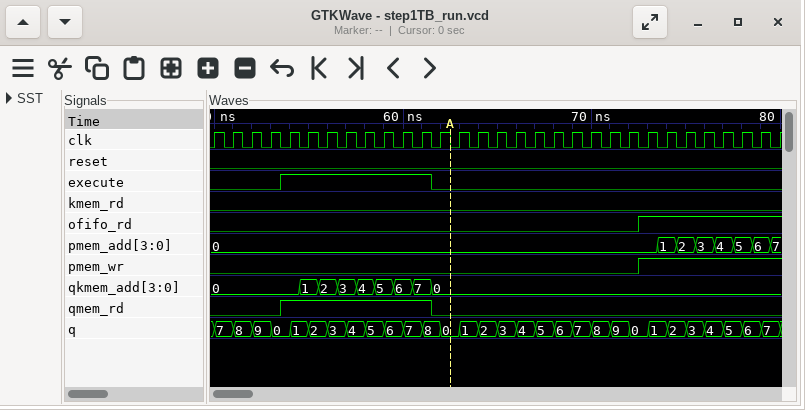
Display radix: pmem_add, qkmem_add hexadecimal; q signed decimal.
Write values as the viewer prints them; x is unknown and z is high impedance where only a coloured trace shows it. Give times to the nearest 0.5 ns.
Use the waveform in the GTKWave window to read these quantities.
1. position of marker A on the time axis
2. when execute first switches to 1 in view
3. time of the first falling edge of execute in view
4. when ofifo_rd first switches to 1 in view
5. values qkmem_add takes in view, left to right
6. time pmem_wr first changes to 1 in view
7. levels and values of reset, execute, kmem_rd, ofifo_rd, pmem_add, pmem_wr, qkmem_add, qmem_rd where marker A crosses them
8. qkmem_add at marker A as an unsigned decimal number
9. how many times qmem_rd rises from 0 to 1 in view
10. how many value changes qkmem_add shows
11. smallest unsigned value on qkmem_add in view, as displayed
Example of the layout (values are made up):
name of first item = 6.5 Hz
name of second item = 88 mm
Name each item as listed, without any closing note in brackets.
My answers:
position of marker A on the time axis = 62.5 ns
when execute first switches to 1 in view = 53.5 ns
time of the first falling edge of execute in view = 61.5 ns
when ofifo_rd first switches to 1 in view = 72.5 ns
values qkmem_add takes in view, left to right = 0, 1, 2, 3, 4, 5, 6, 7, 0
time pmem_wr first changes to 1 in view = 72.5 ns
levels and values of reset, execute, kmem_rd, ofifo_rd, pmem_add, pmem_wr, qkmem_add, qmem_rd where marker A crosses them = reset=0, execute=0, kmem_rd=0, ofifo_rd=0, pmem_add=0, pmem_wr=0, qkmem_add=0, qmem_rd=0
qkmem_add at marker A as an unsigned decimal number = 0
how many times qmem_rd rises from 0 to 1 in view = 1
how many value changes qkmem_add shows = 8
smallest unsigned value on qkmem_add in view, as displayed = 0
